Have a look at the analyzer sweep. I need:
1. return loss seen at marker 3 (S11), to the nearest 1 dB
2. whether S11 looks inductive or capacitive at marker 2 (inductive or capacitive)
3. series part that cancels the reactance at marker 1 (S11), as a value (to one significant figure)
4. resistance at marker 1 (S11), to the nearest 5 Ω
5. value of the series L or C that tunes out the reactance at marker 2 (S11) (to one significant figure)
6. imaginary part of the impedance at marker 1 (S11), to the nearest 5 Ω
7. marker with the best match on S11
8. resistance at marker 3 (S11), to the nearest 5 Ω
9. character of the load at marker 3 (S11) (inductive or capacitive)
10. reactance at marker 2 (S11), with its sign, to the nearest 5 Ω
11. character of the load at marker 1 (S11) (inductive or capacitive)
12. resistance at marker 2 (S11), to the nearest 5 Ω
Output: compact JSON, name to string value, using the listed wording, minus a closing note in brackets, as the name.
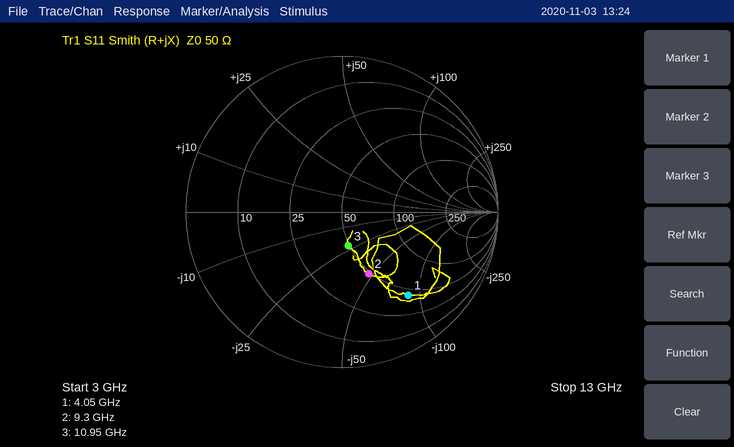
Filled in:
{"return loss seen at marker 3 (S11), to the nearest 1 dB": "13 dB", "whether S11 looks inductive or capacitive at marker 2": "capacitive", "series part that cancels the reactance at marker 1 (S11), as a value": "3 nH", "resistance at marker 1 (S11), to the nearest 5 Ω": "45 Ω", "value of the series L or C that tunes out the reactance at marker 2 (S11)": "800 pH", "imaginary part of the impedance at marker 1 (S11), to the nearest 5 Ω": "-85 Ω", "marker with the best match on S11": "marker 3", "resistance at marker 3 (S11), to the nearest 5 Ω": "50 Ω", "character of the load at marker 3 (S11)": "capacitive", "reactance at marker 2 (S11), with its sign, to the nearest 5 Ω": "-45 Ω", "character of the load at marker 1 (S11)": "capacitive", "resistance at marker 2 (S11), to the nearest 5 Ω": "50 Ω"}
